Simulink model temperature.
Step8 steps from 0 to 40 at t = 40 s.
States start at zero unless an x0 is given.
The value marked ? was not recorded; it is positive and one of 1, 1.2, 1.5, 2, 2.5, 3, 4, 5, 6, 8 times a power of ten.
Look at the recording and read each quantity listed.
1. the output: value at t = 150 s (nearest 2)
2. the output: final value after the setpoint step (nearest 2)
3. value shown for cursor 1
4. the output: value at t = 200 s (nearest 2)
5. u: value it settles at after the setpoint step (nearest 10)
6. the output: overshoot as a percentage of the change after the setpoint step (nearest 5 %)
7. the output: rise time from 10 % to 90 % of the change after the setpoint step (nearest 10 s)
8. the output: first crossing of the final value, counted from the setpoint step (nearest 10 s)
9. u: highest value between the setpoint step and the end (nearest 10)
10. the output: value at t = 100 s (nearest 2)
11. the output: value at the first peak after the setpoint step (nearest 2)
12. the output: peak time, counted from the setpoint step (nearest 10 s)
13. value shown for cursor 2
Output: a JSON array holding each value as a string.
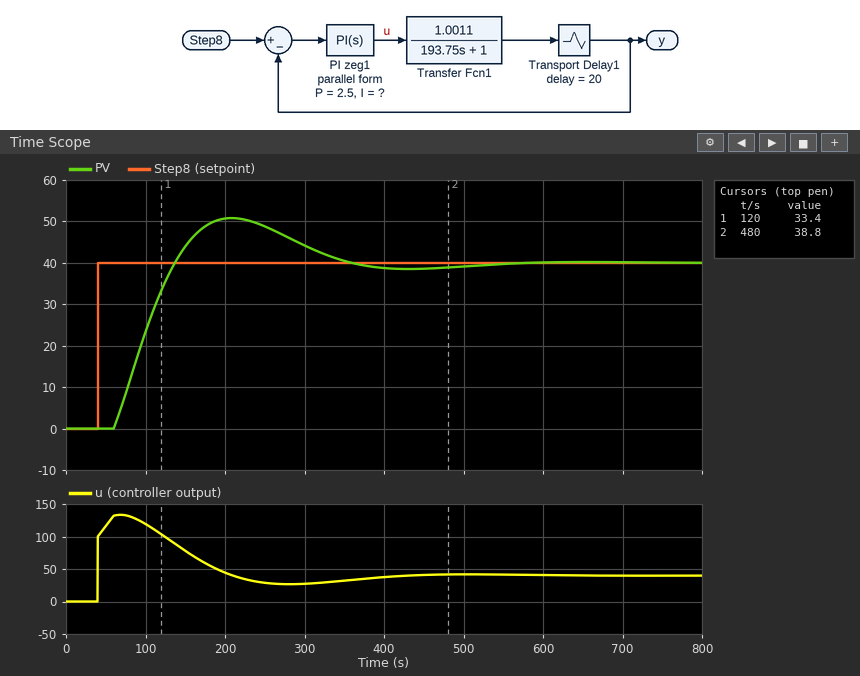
["44", "40", "33.4", "50", "40", "25 %", "60 s", "100 s", "130", "24", "50", "170 s", "38.8"]
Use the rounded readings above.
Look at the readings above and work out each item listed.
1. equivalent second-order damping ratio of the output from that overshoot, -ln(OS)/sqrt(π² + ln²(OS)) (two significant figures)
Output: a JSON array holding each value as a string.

["0.40"]
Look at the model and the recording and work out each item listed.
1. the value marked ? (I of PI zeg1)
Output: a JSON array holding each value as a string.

["0.04"]
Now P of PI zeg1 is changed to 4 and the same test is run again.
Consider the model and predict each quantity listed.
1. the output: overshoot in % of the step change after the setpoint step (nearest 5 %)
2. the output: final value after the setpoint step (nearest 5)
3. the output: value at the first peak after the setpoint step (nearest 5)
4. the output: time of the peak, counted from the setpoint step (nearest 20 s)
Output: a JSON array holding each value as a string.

["15 %", "40", "45", "120 s"]
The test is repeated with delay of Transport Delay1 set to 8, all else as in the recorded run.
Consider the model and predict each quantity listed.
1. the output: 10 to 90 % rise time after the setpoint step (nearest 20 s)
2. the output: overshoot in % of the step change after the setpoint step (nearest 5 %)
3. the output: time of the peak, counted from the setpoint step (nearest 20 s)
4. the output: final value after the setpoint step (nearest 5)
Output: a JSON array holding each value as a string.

["80 s", "20 %", "180 s", "40"]
